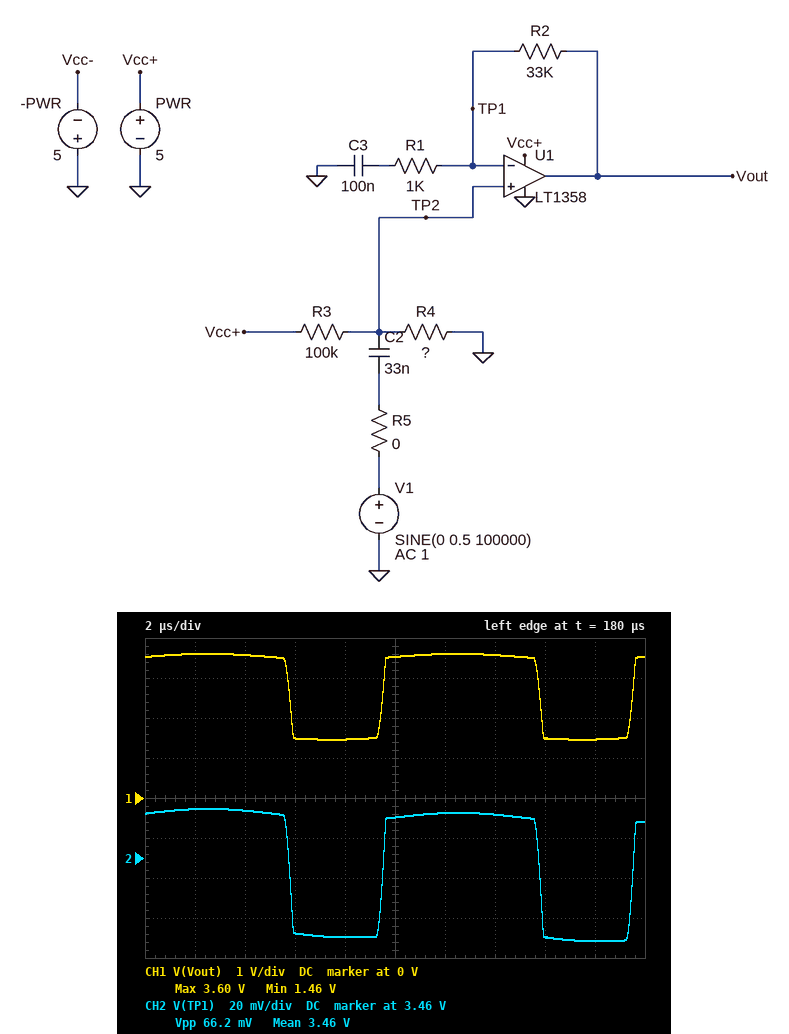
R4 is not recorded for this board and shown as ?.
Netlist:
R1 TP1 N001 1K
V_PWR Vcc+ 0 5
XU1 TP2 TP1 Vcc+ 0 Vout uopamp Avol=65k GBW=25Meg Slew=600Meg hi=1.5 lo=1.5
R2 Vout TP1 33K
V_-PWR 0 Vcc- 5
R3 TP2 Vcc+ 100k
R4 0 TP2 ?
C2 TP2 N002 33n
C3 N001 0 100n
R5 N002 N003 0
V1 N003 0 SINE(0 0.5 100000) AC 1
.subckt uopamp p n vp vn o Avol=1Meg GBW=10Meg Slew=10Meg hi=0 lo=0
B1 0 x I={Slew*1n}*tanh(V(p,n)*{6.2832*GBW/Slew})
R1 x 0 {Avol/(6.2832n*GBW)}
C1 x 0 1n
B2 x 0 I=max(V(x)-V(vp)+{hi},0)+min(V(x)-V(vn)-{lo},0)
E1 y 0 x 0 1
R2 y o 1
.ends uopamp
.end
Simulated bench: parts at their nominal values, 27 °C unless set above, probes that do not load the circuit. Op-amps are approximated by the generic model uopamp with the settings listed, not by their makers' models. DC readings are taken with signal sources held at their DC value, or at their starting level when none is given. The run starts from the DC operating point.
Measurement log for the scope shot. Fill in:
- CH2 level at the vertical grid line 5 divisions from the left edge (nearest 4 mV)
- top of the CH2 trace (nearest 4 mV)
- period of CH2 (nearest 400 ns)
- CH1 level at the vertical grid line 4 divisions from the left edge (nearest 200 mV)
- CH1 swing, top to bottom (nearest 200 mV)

3.480 V
3.484 V
10.0 µs
1.4 V
2.2 V
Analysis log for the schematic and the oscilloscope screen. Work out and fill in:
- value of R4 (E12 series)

270 kΩ
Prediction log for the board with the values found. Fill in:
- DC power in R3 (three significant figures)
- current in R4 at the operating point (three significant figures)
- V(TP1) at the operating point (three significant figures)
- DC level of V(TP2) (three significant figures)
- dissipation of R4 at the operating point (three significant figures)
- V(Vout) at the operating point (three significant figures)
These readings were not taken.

18.3 µW
13.5 µA
3.52 V
3.65 V
49.3 µW
3.52 V
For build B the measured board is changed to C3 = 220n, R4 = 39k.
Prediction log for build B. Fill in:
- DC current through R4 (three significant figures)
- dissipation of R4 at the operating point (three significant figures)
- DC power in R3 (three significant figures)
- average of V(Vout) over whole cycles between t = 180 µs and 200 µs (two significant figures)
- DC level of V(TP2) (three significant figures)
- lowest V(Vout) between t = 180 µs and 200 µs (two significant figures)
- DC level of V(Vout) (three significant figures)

36.0 µA
50.5 µW
129 µW
2.3 V
1.40 V
1.4 V
1.49 V
